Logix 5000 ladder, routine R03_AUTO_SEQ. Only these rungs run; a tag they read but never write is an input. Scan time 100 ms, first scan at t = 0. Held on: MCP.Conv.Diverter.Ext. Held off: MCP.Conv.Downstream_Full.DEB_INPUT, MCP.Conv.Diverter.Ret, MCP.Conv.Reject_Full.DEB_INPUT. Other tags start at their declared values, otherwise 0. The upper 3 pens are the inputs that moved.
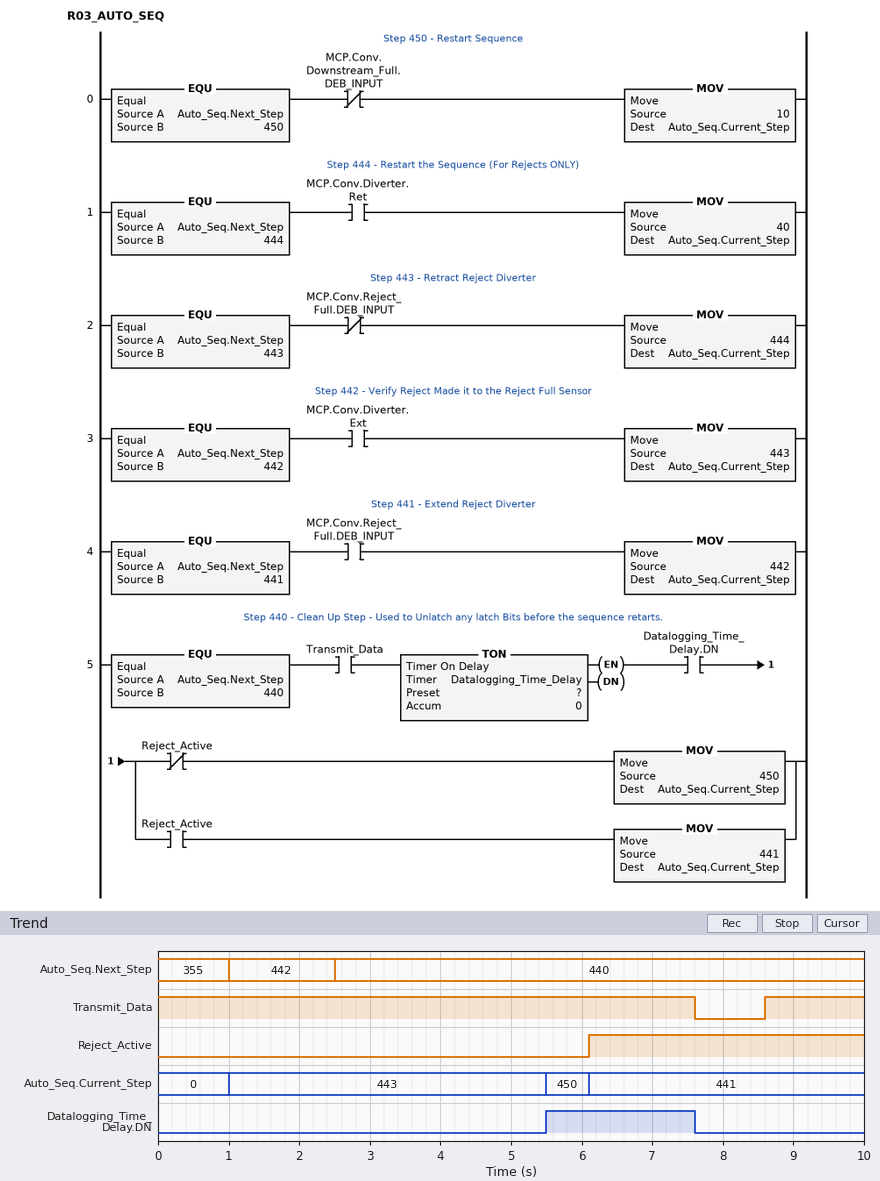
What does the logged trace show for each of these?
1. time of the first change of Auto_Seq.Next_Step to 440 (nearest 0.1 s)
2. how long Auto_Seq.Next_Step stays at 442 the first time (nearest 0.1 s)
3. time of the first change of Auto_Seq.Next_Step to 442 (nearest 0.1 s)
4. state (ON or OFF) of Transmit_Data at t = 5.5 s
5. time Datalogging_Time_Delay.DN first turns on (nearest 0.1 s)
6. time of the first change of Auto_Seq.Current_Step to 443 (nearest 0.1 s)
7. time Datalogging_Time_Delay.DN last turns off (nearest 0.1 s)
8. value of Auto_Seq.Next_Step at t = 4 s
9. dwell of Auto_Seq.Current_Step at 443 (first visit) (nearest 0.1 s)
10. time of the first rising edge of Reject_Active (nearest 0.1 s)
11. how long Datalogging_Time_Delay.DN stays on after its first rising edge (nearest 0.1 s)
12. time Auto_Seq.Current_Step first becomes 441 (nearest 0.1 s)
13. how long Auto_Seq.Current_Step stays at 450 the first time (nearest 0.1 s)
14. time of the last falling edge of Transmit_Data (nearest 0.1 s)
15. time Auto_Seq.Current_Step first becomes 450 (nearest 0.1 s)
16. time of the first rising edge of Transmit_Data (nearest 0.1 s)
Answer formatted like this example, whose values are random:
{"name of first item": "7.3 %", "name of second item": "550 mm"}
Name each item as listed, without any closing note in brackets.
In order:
{"time of the first change of Auto_Seq.Next_Step to 440": "2.5 s", "how long Auto_Seq.Next_Step stays at 442 the first time": "1.5 s", "time of the first change of Auto_Seq.Next_Step to 442": "1.0 s", "state (ON or OFF) of Transmit_Data at t = 5.5 s": "ON", "time Datalogging_Time_Delay.DN first turns on": "5.5 s", "time of the first change of Auto_Seq.Current_Step to 443": "1.0 s", "time Datalogging_Time_Delay.DN last turns off": "7.6 s", "value of Auto_Seq.Next_Step at t = 4 s": "440", "dwell of Auto_Seq.Current_Step at 443 (first visit)": "4.5 s", "time of the first rising edge of Reject_Active": "6.1 s", "how long Datalogging_Time_Delay.DN stays on after its first rising edge": "2.1 s", "time Auto_Seq.Current_Step first becomes 441": "6.1 s", "how long Auto_Seq.Current_Step stays at 450 the first time": "0.6 s", "time of the last falling edge of Transmit_Data": "7.6 s", "time Auto_Seq.Current_Step first becomes 450": "5.5 s", "time of the first rising edge of Transmit_Data": "8.6 s"}
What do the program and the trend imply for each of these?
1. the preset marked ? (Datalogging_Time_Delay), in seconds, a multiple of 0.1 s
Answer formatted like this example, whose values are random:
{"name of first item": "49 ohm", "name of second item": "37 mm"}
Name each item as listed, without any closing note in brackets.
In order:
{"the preset marked ? (Datalogging_Time_Delay), in seconds, a multiple of 0.1 s": "3.0 s"}
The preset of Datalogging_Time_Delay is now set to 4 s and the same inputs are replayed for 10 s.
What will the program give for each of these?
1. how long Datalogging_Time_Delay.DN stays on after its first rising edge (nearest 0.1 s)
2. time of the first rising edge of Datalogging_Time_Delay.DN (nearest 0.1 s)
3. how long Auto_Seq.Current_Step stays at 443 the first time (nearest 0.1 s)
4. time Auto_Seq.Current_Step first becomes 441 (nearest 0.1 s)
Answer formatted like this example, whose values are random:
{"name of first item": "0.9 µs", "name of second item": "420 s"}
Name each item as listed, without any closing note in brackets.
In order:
{"how long Datalogging_Time_Delay.DN stays on after its first rising edge": "1.1 s", "time of the first rising edge of Datalogging_Time_Delay.DN": "6.5 s", "how long Auto_Seq.Current_Step stays at 443 the first time": "5.5 s", "time Auto_Seq.Current_Step first becomes 441": "6.5 s"}
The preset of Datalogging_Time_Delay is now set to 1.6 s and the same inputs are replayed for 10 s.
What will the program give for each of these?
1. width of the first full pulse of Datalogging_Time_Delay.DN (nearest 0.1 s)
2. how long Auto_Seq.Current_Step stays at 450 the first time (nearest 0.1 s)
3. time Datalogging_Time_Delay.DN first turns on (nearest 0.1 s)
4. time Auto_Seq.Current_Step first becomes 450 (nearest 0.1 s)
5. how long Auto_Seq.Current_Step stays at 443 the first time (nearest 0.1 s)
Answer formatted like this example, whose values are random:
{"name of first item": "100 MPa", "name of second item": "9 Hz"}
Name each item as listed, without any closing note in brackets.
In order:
{"width of the first full pulse of Datalogging_Time_Delay.DN": "3.5 s", "how long Auto_Seq.Current_Step stays at 450 the first time": "2.0 s", "time Datalogging_Time_Delay.DN first turns on": "4.1 s", "time Auto_Seq.Current_Step first becomes 450": "4.1 s", "how long Auto_Seq.Current_Step stays at 443 the first time": "3.1 s"}
